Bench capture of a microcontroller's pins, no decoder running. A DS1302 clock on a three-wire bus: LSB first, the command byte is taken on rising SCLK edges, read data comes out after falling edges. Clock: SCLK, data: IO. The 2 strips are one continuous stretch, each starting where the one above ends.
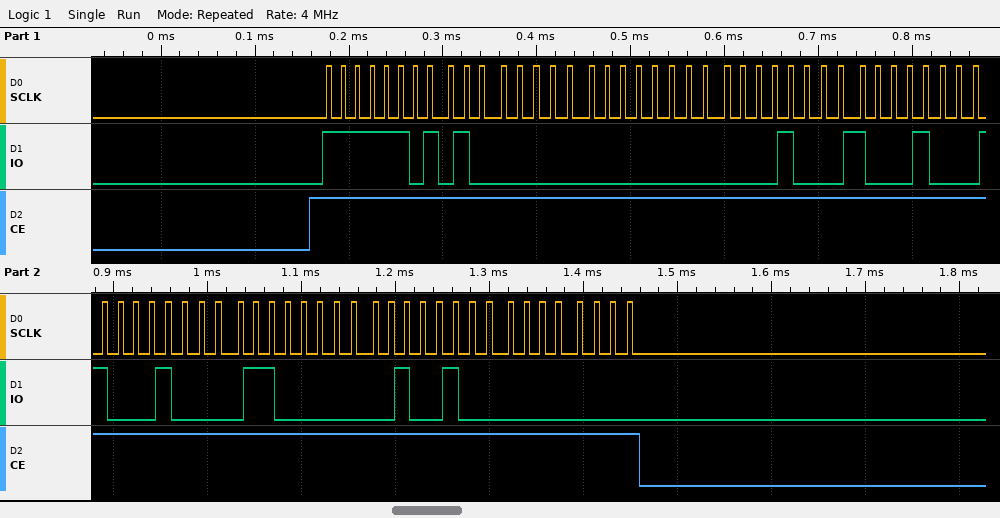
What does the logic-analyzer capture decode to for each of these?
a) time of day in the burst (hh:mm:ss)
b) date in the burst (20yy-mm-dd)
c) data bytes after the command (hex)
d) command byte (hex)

10:00:02
2024-11-11
02 00 10 11 11 06 24 00
0xBF
